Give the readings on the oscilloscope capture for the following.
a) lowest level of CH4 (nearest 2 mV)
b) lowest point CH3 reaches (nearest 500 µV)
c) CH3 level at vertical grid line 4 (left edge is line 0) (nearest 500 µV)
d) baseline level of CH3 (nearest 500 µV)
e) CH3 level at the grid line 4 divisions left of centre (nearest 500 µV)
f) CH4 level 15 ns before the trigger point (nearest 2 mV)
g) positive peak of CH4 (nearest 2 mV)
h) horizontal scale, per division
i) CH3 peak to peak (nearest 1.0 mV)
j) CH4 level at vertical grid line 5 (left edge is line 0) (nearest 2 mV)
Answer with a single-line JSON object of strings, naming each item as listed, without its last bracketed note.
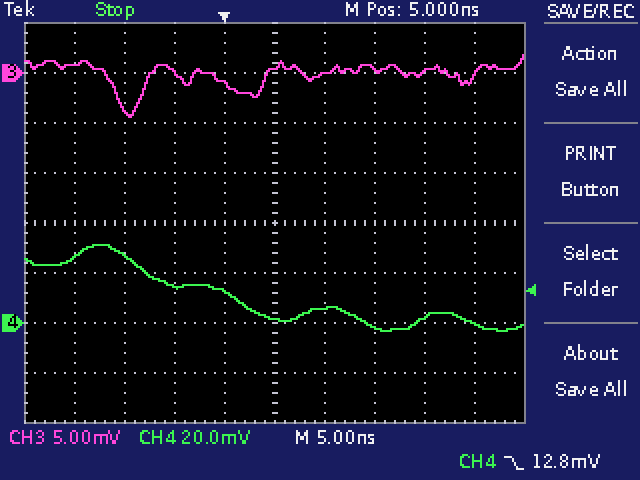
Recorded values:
{"lowest level of CH4": "-4 mV", "lowest point CH3 reaches": "-4.5 mV", "CH3 level at vertical grid line 4 (left edge is line 0)": "-1.0 mV", "baseline level of CH3": "500 µV", "CH3 level at the grid line 4 divisions left of centre": "1.0 mV", "CH4 level 15 ns before the trigger point": "26 mV", "positive peak of CH4": "32 mV", "horizontal scale, per division": "5 ns", "CH3 peak to peak": "6.0 mV", "CH4 level at vertical grid line 5 (left edge is line 0)": "2 mV"}
